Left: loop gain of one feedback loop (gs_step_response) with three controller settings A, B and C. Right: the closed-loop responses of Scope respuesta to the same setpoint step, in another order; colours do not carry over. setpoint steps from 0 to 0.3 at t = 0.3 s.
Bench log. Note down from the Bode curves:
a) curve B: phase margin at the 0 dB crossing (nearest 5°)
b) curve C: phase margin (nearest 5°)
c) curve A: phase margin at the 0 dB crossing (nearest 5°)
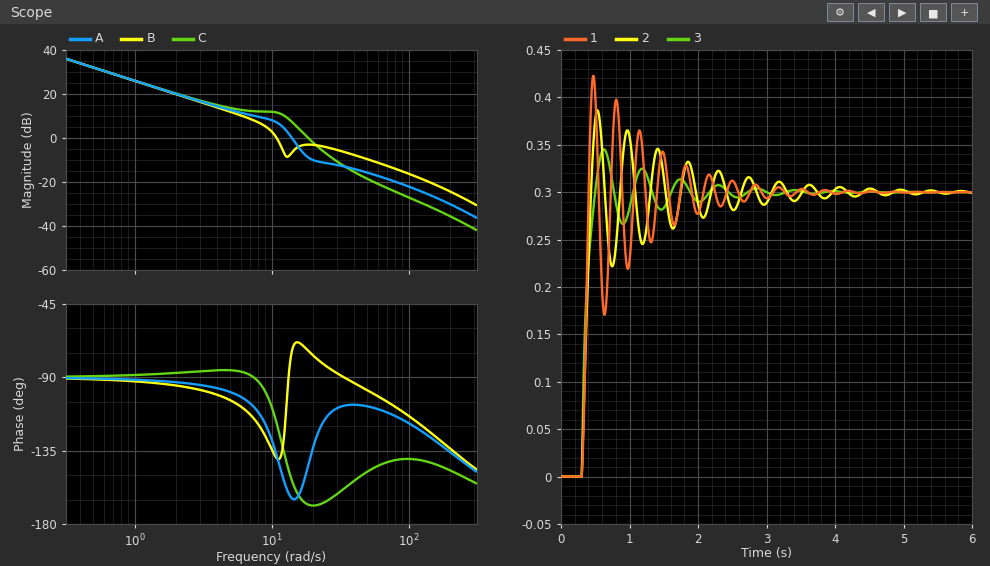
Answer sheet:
40°
10°
15°
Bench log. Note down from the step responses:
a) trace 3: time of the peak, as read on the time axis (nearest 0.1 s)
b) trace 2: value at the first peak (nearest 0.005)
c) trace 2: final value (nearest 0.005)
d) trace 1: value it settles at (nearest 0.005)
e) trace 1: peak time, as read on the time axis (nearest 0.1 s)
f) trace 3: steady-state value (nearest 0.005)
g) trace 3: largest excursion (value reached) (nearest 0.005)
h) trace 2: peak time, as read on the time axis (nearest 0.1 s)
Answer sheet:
0.6 s
0.385
0.300
0.300
0.5 s
0.300
0.345
0.5 s
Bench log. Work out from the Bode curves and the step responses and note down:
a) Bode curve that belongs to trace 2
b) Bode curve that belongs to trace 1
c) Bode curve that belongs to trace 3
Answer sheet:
A
C
B
